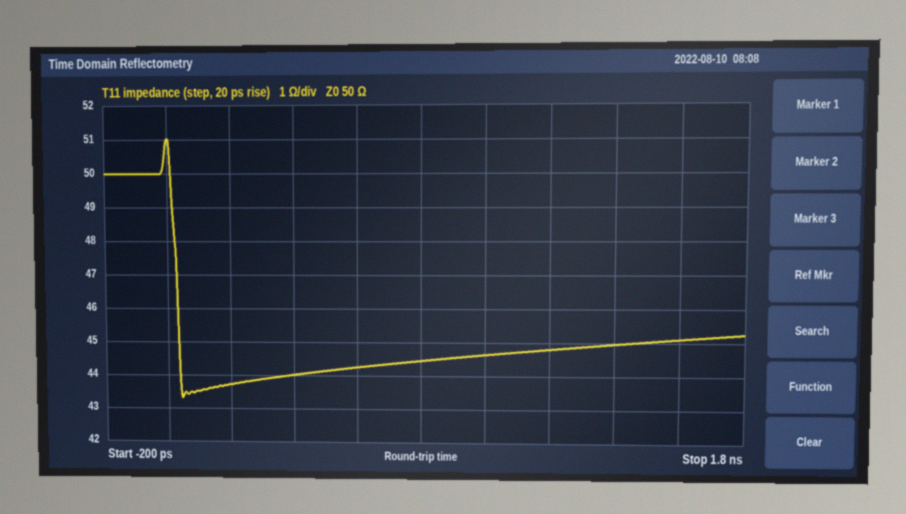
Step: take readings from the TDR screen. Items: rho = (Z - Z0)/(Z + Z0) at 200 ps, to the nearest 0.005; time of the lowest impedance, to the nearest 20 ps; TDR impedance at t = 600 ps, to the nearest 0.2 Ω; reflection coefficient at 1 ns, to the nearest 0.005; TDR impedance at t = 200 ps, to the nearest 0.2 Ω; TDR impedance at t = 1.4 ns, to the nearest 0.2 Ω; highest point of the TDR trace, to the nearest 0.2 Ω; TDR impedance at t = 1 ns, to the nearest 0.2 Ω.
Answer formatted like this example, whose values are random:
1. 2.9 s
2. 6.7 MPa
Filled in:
1. -0.065
2. 40 ps
3. 44.2 Ω
4. -0.055
5. 43.8 Ω
6. 45.0 Ω
7. 51.0 Ω
8. 44.6 Ω
